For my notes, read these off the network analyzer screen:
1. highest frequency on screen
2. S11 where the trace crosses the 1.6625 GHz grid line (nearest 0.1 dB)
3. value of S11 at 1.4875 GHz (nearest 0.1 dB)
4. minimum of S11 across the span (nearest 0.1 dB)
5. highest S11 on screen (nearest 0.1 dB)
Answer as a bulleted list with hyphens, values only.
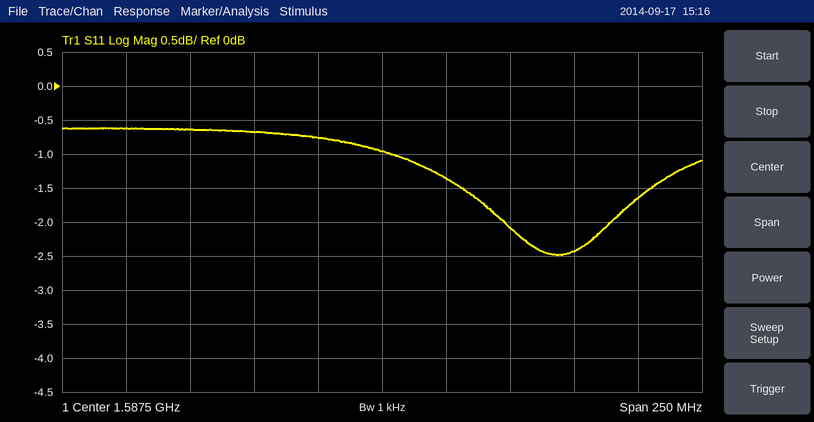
- 1.7125 GHz
- -2.4 dB
- -0.6 dB
- -2.5 dB
- -0.6 dB
